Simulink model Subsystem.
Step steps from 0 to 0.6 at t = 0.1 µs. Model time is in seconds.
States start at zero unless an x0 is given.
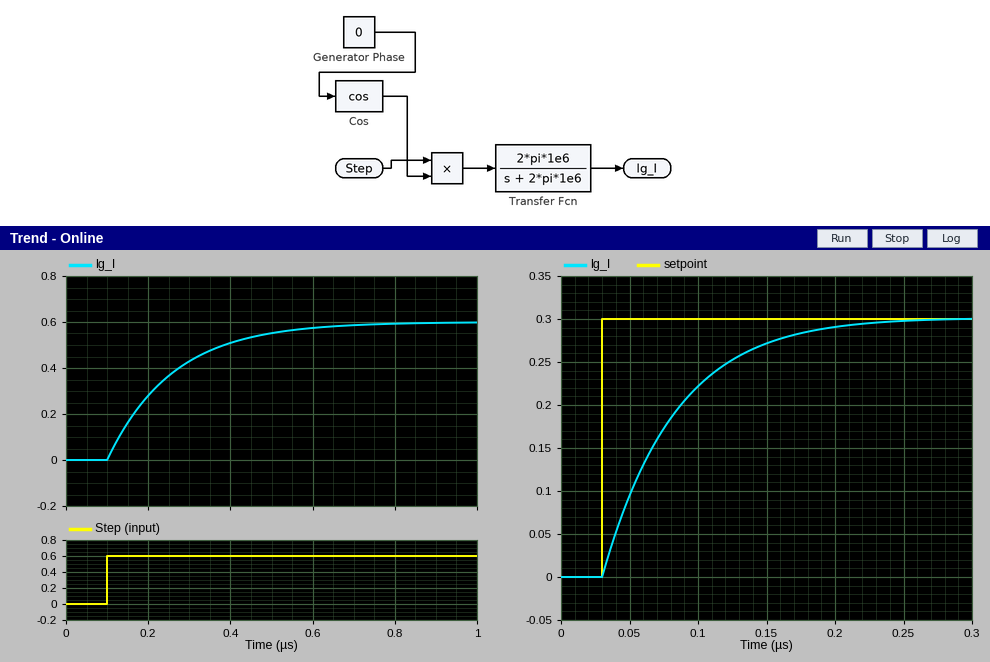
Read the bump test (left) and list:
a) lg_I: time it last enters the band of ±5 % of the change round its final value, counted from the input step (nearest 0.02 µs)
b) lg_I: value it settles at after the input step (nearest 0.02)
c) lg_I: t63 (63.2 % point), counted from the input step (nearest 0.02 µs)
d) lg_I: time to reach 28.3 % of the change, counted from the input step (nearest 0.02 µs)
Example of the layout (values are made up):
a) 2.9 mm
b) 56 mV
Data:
a) 0.48 µs
b) 0.60
c) 0.16 µs
d) 0.06 µs
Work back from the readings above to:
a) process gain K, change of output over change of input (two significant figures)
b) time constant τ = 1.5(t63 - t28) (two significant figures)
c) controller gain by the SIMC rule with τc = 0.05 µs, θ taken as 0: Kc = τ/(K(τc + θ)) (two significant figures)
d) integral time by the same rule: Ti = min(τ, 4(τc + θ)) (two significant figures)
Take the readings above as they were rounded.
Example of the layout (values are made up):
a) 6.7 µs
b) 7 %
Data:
a) 1.0
b) 0.15 µs
c) 3.0
d) 0.15 µs
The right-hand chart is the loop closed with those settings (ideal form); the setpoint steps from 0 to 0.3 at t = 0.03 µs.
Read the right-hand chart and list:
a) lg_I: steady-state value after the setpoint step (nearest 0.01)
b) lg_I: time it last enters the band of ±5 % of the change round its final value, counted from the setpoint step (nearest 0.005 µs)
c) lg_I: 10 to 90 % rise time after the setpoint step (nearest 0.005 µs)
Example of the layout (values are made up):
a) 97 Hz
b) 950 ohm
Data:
a) 0.30
b) 0.150 µs
c) 0.110 µs
